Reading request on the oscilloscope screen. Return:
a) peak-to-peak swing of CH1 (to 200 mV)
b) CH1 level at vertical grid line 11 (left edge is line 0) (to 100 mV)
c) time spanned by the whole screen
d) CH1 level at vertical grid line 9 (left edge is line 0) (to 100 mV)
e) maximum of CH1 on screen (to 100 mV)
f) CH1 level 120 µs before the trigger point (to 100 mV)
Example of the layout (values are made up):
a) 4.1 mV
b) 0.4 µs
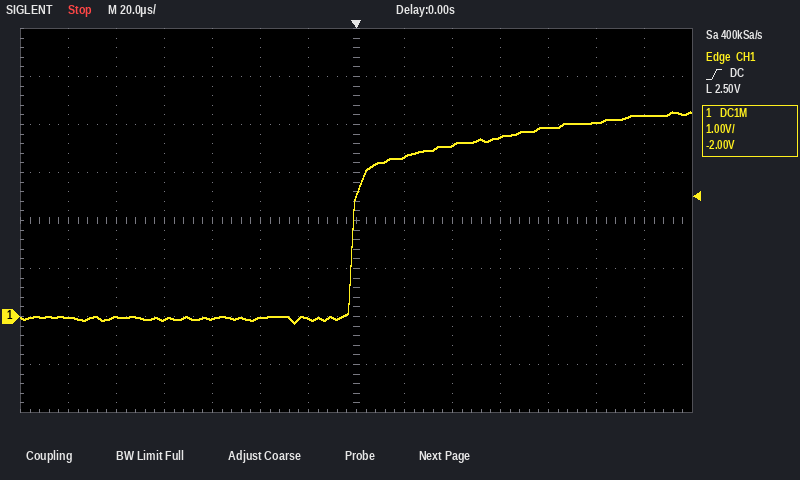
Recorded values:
a) 4.4 V
b) 3.9 V
c) 280 µs
d) 3.6 V
e) 4.3 V
f) 0.0 V
